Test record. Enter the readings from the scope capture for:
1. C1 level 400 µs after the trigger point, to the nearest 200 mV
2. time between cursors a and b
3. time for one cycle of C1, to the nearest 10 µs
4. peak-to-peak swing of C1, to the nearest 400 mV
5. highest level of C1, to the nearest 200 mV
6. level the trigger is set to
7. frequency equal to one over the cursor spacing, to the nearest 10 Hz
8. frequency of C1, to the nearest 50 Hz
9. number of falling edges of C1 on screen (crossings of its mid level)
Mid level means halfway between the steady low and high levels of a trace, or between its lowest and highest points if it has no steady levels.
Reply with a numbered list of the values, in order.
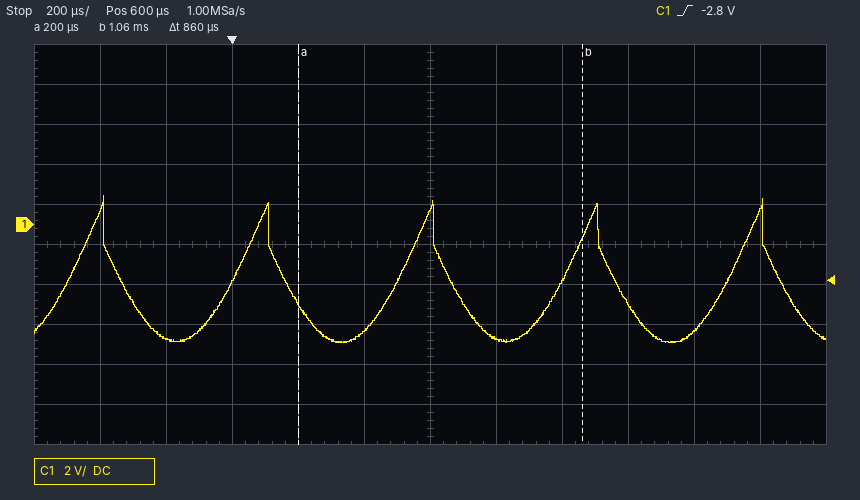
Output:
1. -5.4 V
2. 860 µs
3. 500 µs
4. 7.2 V
5. 1.4 V
6. -2.8 V
7. 1.16 kHz
8. 2.00 kHz
9. 5
